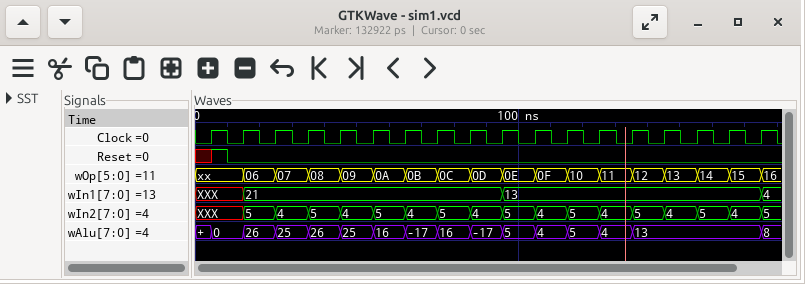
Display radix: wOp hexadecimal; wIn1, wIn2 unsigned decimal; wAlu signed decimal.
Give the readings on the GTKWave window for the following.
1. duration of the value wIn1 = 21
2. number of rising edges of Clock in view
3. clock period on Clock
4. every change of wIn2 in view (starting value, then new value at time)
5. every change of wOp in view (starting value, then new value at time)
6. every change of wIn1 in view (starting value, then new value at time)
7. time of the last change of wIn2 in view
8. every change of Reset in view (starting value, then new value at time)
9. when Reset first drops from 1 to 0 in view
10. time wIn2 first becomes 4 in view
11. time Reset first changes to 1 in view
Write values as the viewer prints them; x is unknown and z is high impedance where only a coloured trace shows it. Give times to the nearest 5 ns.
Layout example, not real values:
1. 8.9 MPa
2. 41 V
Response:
1. 80 ns
2. 18
3. 10 ns
4. XXX, 5 at 15 ns, 4 at 25 ns, 5 at 35 ns, 4 at 45 ns, 5 at 55 ns, 4 at 65 ns, 5 at 75 ns, 4 at 85 ns, 5 at 95 ns, 4 at 105 ns, 5 at 115 ns, 4 at 125 ns, 5 at 135 ns, 4 at 145 ns, 5 at 155 ns, 4 at 165 ns, 5 at 175 ns
5. xx, 06 at 15 ns, 07 at 25 ns, 08 at 35 ns, 09 at 45 ns, 0A at 55 ns, 0B at 65 ns, 0C at 75 ns, 0D at 85 ns, 0E at 95 ns, 0F at 105 ns, 10 at 115 ns, 11 at 125 ns, 12 at 135 ns, 13 at 145 ns, 14 at 155 ns, 15 at 165 ns, 16 at 175 ns
6. XXX, 21 at 15 ns, 13 at 95 ns, 4 at 175 ns
7. 175 ns
8. x, 1 at 5 ns, 0 at 10 ns
9. 10 ns
10. 25 ns
11. 5 ns
